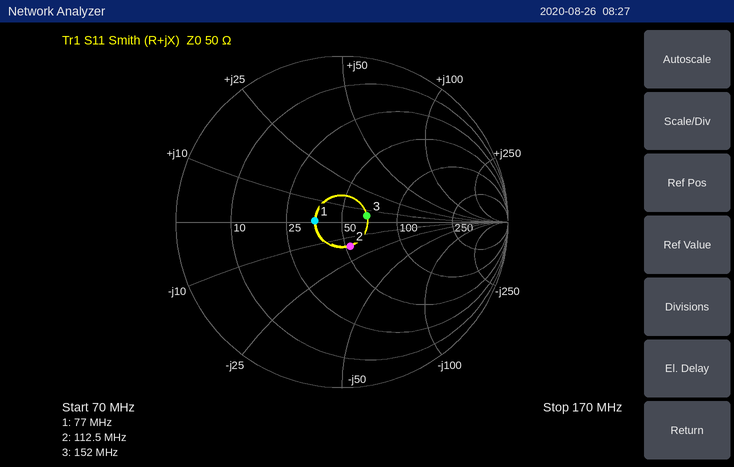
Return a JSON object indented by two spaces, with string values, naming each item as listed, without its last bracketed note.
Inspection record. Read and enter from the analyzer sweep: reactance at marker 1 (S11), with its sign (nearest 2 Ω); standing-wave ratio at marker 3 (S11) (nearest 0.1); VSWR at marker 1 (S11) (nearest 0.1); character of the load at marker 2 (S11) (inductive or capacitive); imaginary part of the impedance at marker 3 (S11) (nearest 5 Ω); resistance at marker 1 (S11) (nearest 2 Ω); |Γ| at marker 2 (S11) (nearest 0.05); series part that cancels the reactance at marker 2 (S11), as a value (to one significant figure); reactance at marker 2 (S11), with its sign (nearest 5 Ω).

{
  "reactance at marker 1 (S11), with its sign": "0 Ω",
  "standing-wave ratio at marker 3 (S11)": "1.4",
  "VSWR at marker 1 (S11)": "1.4",
  "character of the load at marker 2 (S11)": "capacitive",
  "imaginary part of the impedance at marker 3 (S11)": "+5 Ω",
  "resistance at marker 1 (S11)": "36 Ω",
  "|Γ| at marker 2 (S11)": "0.15",
  "series part that cancels the reactance at marker 2 (S11), as a value": "20 nH",
  "reactance at marker 2 (S11), with its sign": "-15 Ω"
}
